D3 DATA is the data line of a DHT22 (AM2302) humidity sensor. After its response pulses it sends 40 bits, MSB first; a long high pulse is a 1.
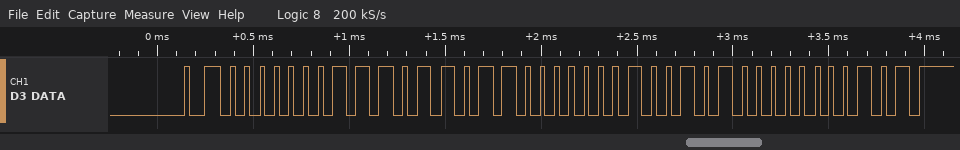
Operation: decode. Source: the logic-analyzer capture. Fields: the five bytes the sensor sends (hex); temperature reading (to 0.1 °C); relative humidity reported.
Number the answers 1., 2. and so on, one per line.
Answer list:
1. 01 DB 01 28 05
2. 29.6 °C
3. 47.5 %
